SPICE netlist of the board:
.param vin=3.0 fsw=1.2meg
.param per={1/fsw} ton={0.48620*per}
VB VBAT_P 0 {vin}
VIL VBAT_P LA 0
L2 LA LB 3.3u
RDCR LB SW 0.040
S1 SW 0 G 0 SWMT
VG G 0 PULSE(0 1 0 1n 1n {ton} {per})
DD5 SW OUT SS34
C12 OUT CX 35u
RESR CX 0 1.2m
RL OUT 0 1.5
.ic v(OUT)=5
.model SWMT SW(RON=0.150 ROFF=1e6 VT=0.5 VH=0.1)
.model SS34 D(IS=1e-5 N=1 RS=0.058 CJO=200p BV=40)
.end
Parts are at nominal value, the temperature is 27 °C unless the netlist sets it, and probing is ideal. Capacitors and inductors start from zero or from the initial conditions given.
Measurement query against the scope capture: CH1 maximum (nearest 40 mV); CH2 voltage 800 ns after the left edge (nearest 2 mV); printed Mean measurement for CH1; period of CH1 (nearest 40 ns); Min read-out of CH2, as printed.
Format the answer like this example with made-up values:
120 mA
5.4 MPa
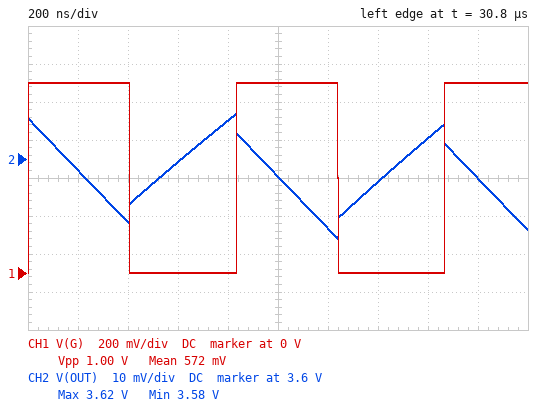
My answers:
1.00 V
3.610 V
572 mV
840 ns
3.58 V
